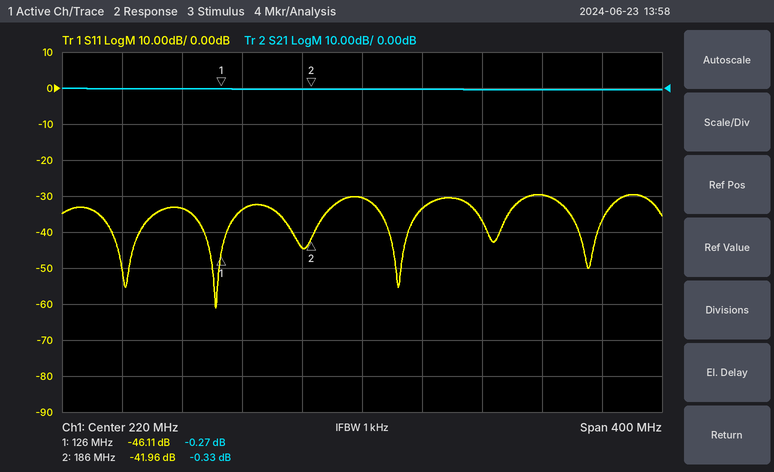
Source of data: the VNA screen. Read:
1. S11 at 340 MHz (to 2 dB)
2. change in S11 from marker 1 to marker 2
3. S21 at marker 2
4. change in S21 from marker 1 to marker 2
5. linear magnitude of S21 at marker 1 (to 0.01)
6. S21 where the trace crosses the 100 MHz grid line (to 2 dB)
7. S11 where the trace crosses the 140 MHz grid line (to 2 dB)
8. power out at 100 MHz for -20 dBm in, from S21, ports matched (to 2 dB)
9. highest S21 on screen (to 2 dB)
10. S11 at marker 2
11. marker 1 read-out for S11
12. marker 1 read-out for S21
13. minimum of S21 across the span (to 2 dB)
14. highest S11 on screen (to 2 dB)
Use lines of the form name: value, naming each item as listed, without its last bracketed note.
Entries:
S11 at 340 MHz: -30 dB
change in S11 from marker 1 to marker 2: 4.15 dB
S21 at marker 2: -0.33 dB
change in S21 from marker 1 to marker 2: -0.06 dB
linear magnitude of S21 at marker 1: 0.97
S21 where the trace crosses the 100 MHz grid line: 0 dB
S11 where the trace crosses the 140 MHz grid line: -34 dB
power out at 100 MHz for -20 dBm in, from S21, ports matched: -20 dBm
highest S21 on screen: 0 dB
S11 at marker 2: -41.96 dB
marker 1 read-out for S11: -46.11 dB
marker 1 read-out for S21: -0.27 dB
minimum of S21 across the span: 0 dB
highest S11 on screen: -30 dB
